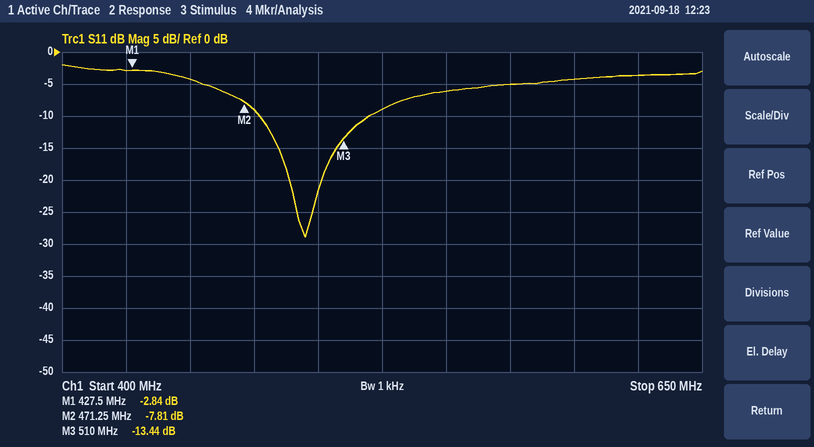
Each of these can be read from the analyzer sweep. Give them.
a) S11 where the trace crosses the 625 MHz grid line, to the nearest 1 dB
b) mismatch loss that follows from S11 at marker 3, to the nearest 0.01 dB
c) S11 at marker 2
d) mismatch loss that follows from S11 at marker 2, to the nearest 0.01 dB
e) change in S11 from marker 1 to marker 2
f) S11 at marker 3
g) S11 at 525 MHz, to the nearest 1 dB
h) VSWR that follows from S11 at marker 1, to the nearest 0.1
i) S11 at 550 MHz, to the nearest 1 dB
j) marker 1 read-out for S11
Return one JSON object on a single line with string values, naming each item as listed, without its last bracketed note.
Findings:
{"S11 where the trace crosses the 625 MHz grid line, to the nearest 1 dB": "-4 dB", "mismatch loss that follows from S11 at marker 3, to the nearest 0.01 dB": "0.20 dB", "S11 at marker 2": "-7.81 dB", "mismatch loss that follows from S11 at marker 2, to the nearest 0.01 dB": "0.79 dB", "change in S11 from marker 1 to marker 2": "-4.97 dB", "S11 at marker 3": "-13.44 dB", "S11 at 525 MHz, to the nearest 1 dB": "-9 dB", "VSWR that follows from S11 at marker 1, to the nearest 0.1": "6.2", "S11 at 550 MHz, to the nearest 1 dB": "-6 dB", "marker 1 read-out for S11": "-2.84 dB"}
